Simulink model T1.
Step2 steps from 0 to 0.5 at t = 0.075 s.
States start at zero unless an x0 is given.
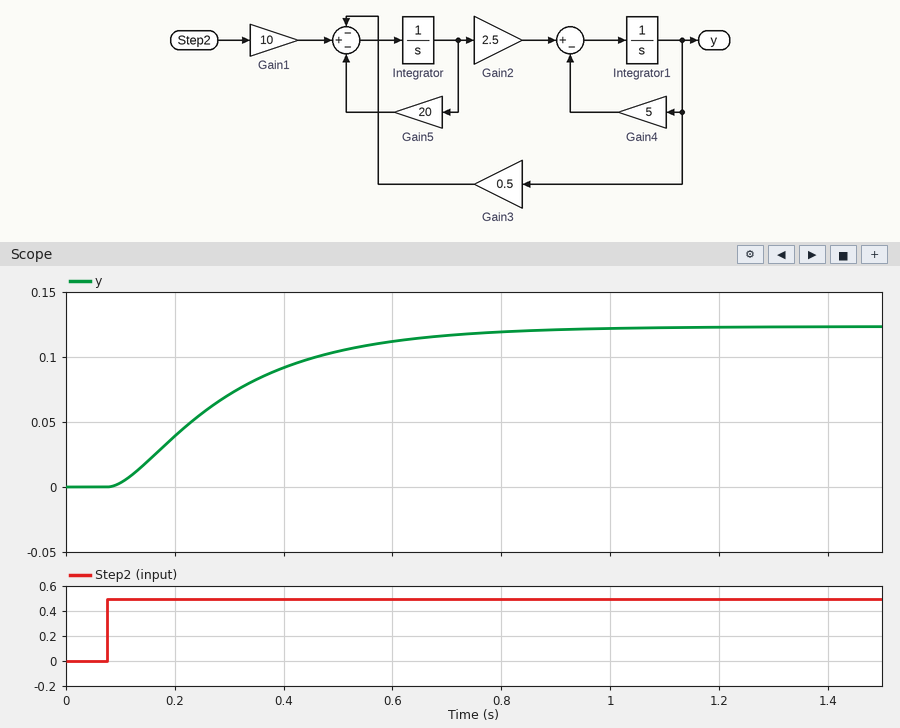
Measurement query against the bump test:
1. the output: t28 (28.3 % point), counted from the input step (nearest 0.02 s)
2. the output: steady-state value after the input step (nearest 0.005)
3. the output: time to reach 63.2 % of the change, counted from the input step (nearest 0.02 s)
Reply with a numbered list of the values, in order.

1. 0.12 s
2. 0.125
3. 0.26 s
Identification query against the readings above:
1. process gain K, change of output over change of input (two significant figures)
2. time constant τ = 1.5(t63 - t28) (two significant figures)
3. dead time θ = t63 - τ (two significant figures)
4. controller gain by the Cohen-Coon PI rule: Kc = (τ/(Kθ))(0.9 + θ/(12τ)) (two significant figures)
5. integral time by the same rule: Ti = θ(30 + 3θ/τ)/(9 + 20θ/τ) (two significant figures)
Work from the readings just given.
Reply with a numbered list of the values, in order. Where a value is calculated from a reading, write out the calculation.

1. (0.125 - 0) / 0.5 = 0.25
2. 1.5 × (0.26 - 0.12) = 0.21 s
3. 0.26 - 0.21 = 0.050 s
4. 0.21 / (0.25 × 0.05) × (0.9 + 0.05 / (12 × 0.21)) = 15
5. 0.05 × (30 + 3 × 0.05 / 0.21) / (9 + 20 × 0.05 / 0.21) = 0.11 s
